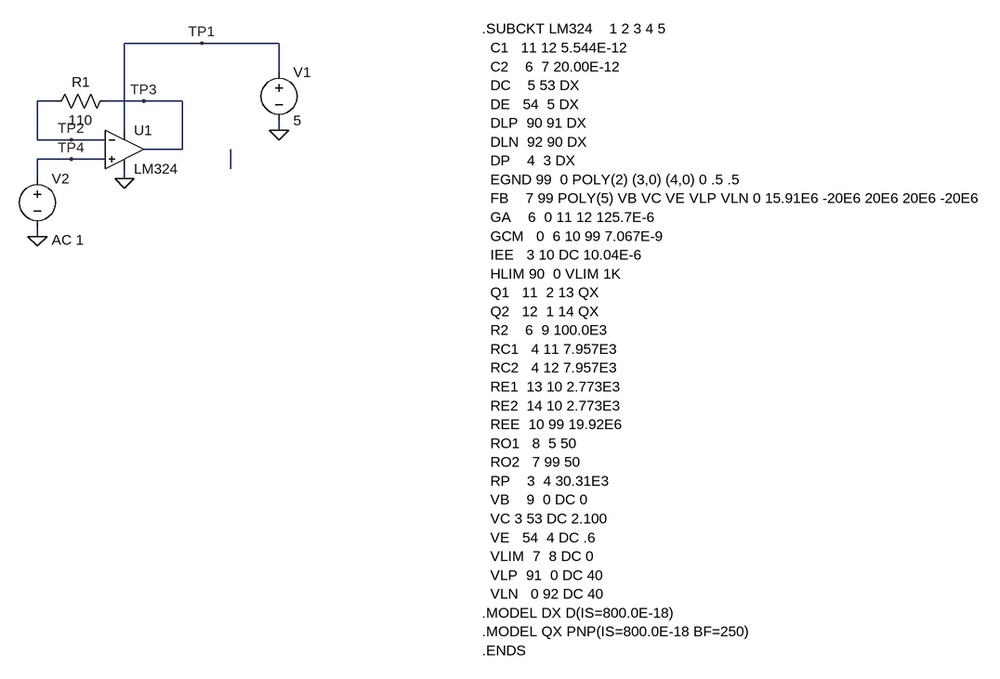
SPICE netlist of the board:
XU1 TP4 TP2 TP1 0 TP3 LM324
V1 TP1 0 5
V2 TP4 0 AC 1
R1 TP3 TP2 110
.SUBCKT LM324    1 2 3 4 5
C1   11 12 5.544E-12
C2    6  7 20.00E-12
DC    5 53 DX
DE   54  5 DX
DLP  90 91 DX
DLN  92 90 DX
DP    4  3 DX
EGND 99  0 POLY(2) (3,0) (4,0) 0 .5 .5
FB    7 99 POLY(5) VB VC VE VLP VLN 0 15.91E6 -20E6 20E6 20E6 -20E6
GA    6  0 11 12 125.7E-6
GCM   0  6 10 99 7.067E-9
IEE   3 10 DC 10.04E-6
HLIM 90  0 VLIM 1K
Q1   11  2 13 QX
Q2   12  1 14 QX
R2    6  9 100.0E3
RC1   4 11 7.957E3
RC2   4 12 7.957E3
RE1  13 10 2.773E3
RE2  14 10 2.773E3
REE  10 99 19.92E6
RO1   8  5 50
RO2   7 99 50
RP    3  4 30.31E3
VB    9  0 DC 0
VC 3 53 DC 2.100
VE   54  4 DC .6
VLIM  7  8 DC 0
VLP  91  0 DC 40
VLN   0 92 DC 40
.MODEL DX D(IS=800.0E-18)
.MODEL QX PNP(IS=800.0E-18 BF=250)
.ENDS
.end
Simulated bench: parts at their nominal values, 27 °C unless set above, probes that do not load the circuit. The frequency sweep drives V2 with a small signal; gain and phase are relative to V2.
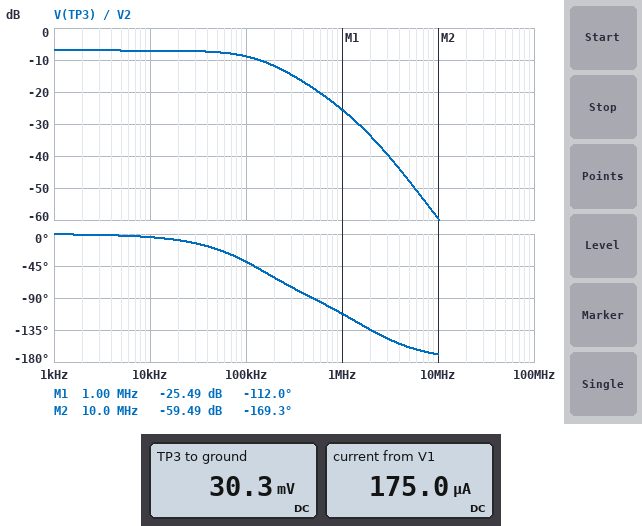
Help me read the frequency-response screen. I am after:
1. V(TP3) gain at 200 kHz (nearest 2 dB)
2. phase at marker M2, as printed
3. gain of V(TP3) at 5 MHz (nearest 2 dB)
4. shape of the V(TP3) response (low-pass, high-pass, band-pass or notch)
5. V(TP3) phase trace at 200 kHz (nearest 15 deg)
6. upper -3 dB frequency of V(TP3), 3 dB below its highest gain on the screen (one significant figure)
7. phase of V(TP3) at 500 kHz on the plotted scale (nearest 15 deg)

-12 dB
-169.3 deg
-48 dB
low-pass
-60 deg
100 kHz
-90 deg
